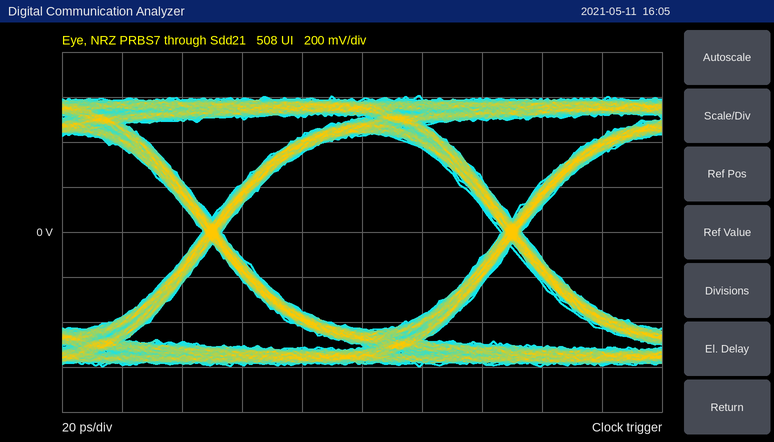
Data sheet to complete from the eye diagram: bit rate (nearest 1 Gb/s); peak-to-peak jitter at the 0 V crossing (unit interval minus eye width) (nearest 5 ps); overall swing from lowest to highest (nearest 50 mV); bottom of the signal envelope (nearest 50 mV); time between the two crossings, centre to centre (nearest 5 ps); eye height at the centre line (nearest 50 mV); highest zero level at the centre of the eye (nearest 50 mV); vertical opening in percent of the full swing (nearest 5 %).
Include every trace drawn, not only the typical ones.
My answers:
10 Gb/s
5 ps
1.20 V
-600 mV
100 ps
850 mV
-450 mV
70 %
